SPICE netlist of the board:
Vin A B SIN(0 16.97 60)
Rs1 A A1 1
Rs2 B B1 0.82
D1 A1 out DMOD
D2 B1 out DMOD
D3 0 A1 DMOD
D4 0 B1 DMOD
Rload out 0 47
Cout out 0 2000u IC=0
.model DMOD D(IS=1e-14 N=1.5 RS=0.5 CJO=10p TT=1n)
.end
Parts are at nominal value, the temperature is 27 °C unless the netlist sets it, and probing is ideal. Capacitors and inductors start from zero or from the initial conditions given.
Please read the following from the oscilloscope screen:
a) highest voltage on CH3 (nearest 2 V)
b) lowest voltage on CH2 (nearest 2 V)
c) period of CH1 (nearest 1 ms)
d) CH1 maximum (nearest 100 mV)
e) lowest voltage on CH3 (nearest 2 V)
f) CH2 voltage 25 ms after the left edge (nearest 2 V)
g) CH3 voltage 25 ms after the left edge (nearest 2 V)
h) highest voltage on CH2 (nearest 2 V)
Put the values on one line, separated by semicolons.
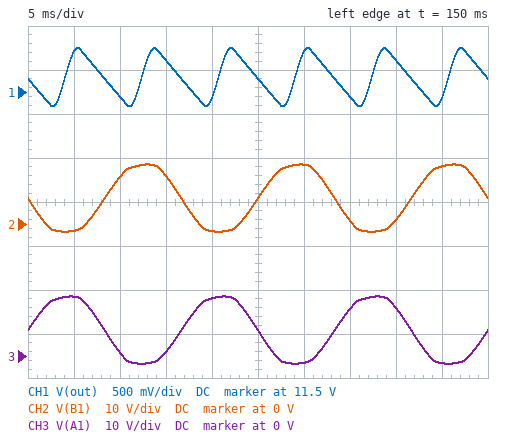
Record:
14 V; -2 V; 8 ms; 12.0 V; -2 V; 6 V; 6 V; 14 V
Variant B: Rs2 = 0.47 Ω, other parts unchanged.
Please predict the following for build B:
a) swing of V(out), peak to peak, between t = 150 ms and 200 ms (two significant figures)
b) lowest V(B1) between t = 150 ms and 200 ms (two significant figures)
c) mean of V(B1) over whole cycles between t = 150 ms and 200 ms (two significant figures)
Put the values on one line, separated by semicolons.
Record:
690 mV; -1.8 V; 5.9 V
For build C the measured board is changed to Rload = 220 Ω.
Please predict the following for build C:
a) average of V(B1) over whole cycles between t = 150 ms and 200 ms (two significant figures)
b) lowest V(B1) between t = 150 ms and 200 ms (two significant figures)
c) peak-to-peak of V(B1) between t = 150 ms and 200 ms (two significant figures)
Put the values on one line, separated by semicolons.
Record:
6.7 V; -1.4 V; 16 V
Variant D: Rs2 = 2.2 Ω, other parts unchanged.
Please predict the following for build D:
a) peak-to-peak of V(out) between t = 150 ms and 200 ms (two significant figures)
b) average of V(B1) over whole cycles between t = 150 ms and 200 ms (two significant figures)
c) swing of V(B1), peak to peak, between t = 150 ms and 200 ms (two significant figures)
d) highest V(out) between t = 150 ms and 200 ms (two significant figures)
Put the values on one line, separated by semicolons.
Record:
590 mV; 5.5 V; 14 V; 11 V
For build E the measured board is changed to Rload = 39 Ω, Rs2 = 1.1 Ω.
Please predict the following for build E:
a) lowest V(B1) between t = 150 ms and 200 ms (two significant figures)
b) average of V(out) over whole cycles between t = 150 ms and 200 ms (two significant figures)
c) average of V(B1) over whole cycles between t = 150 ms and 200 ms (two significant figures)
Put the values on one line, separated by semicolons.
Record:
-1.8 V; 11 V; 5.6 V
